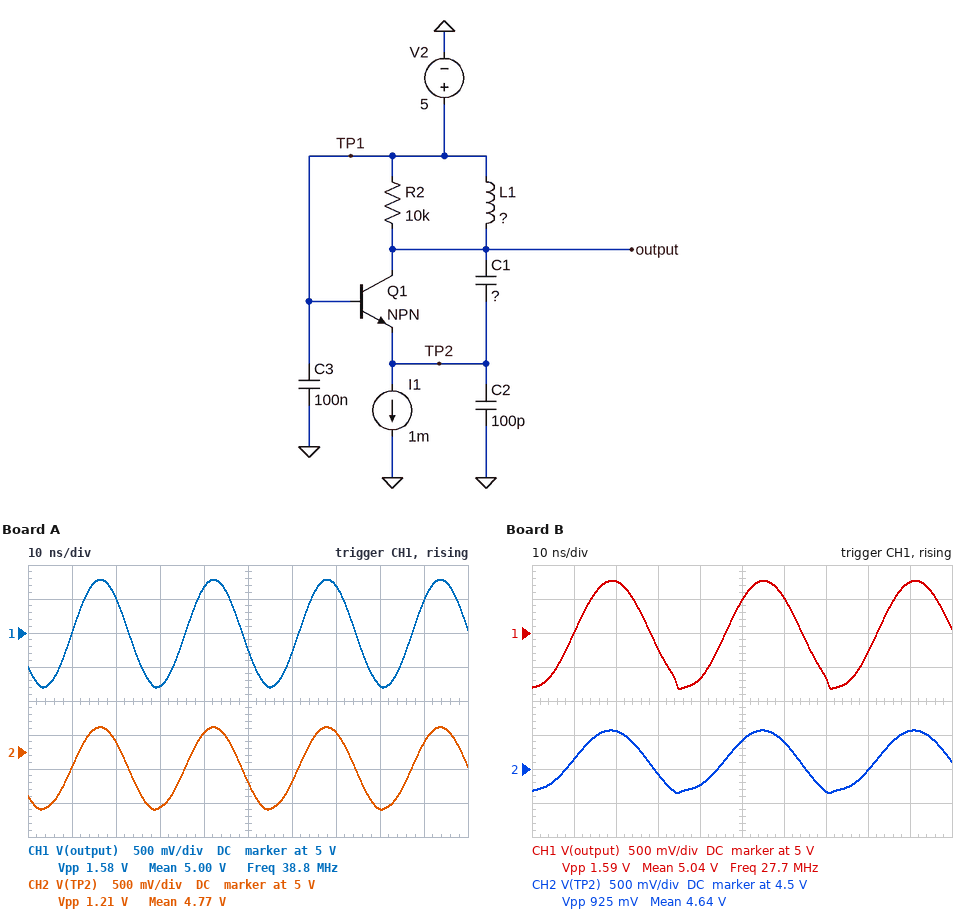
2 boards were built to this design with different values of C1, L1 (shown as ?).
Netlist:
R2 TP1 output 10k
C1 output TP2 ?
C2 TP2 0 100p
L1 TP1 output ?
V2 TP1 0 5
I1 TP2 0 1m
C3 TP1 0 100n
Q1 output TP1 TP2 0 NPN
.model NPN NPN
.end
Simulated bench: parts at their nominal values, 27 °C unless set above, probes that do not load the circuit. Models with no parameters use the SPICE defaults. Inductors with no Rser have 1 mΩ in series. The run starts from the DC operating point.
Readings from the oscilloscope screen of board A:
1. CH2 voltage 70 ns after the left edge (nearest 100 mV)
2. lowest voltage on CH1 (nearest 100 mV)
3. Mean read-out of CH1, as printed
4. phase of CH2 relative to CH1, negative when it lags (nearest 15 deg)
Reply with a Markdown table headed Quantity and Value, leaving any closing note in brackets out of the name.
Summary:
| Quantity | Value |
|---|---|
| CH2 voltage 70 ns after the left edge | 5.3 V |
| lowest voltage on CH1 | 4.2 V |
| Mean read-out of CH1, as printed | 5.00 V |
| phase of CH2 relative to CH1, negative when it lags | 0 deg |
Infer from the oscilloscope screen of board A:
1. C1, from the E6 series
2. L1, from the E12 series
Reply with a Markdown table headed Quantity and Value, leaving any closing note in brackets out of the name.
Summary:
| Quantity | Value |
|---|---|
| C1, from the E6 series | 330 pF |
| L1, from the E12 series | 220 nH |
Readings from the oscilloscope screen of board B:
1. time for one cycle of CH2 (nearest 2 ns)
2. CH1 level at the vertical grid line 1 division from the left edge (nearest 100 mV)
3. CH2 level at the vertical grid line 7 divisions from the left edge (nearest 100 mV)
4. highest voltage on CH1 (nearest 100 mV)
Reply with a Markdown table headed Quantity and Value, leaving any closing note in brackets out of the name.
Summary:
| Quantity | Value |
|---|---|
| time for one cycle of CH2 | 36 ns |
| CH1 level at the vertical grid line 1 division from the left edge | 5.0 V |
| CH2 level at the vertical grid line 7 divisions from the left edge | 4.2 V |
| highest voltage on CH1 | 5.8 V |
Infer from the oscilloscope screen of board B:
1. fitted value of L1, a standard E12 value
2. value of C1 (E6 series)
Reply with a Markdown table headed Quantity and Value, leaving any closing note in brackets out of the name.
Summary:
| Quantity | Value |
|---|---|
| fitted value of L1, a standard E12 value | 560 nH |
| value of C1 | 150 pF |
